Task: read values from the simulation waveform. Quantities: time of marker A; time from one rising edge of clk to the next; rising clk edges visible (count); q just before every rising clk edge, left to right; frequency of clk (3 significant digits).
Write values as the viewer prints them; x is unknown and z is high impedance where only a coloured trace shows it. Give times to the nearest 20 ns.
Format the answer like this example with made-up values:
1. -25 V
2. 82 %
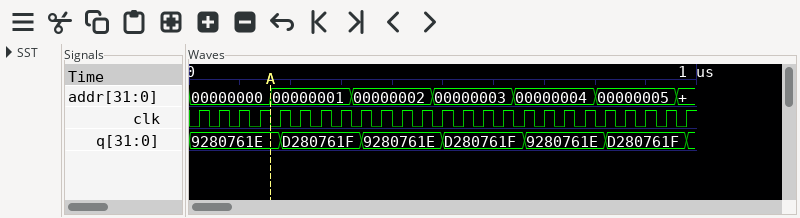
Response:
1. 160 ns
2. 40 ns
3. 25
4. 9280761E, 9280761E, 9280761E, 9280761E, 9280761E, D280761F, D280761F, D280761F, D280761F, 9280761E, 9280761E, 9280761E, 9280761E, D280761F, D280761F, D280761F, D280761F, 9280761E, 9280761E, 9280761E, 9280761E, D280761F, D280761F, D280761F, D280761F
5. 25.0 MHz
